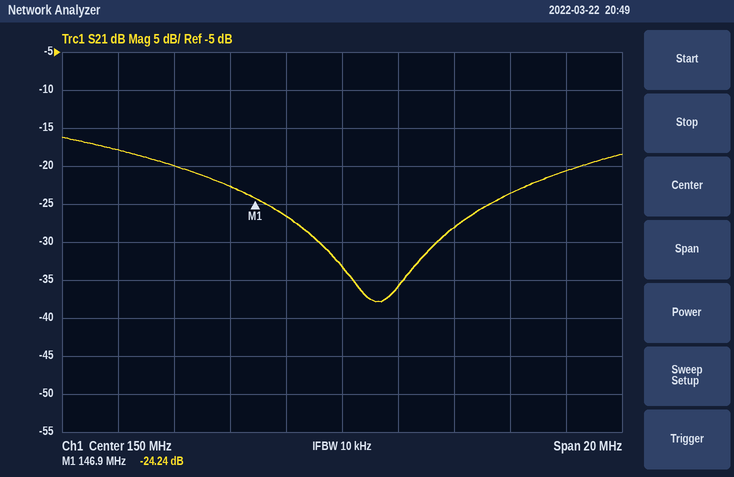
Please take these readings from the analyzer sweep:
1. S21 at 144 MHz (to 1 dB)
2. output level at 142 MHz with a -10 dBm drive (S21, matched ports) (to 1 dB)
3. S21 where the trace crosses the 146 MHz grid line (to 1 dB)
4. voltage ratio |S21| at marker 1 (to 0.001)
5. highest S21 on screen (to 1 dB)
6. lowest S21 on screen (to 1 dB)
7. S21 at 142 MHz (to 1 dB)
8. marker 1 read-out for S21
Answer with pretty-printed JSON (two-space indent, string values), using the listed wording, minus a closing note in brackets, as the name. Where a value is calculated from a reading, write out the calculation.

{
  "S21 at 144 MHz": "-20 dB",
  "output level at 142 MHz with a -10 dBm drive (S21, matched ports)": "-10 dBm + (-18 dB) = -28 dBm",
  "S21 where the trace crosses the 146 MHz grid line": "-23 dB",
  "voltage ratio |S21| at marker 1": "10^(-24.24/20) ≈ 0.061",
  "highest S21 on screen": "-16 dB",
  "lowest S21 on screen": "-38 dB",
  "S21 at 142 MHz": "-18 dB",
  "marker 1 read-out for S21": "-24.24 dB"
}
